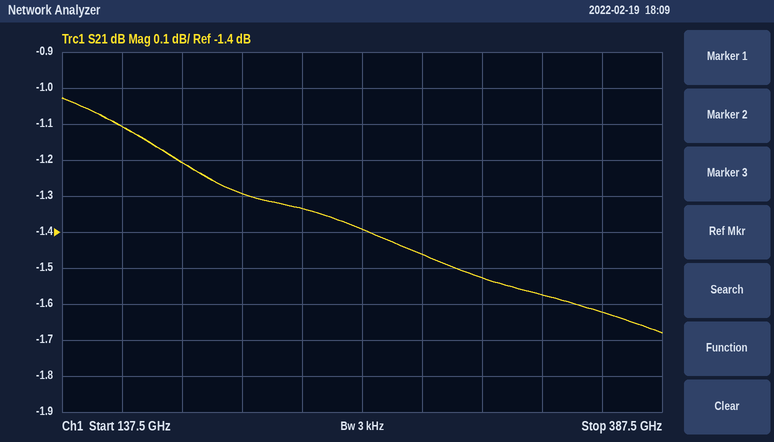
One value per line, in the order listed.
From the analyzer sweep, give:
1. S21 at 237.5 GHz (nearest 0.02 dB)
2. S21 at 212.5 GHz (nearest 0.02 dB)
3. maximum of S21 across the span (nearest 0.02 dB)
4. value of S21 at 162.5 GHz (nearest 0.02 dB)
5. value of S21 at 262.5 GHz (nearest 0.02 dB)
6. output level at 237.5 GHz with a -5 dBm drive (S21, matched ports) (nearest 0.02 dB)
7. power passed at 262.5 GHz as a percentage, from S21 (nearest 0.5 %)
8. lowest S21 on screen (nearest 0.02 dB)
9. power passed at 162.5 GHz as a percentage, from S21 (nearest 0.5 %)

-1.34 dB
-1.30 dB
-1.02 dB
-1.10 dB
-1.40 dB
-6.34 dBm
72.5 %
-1.68 dB
77.5 %
